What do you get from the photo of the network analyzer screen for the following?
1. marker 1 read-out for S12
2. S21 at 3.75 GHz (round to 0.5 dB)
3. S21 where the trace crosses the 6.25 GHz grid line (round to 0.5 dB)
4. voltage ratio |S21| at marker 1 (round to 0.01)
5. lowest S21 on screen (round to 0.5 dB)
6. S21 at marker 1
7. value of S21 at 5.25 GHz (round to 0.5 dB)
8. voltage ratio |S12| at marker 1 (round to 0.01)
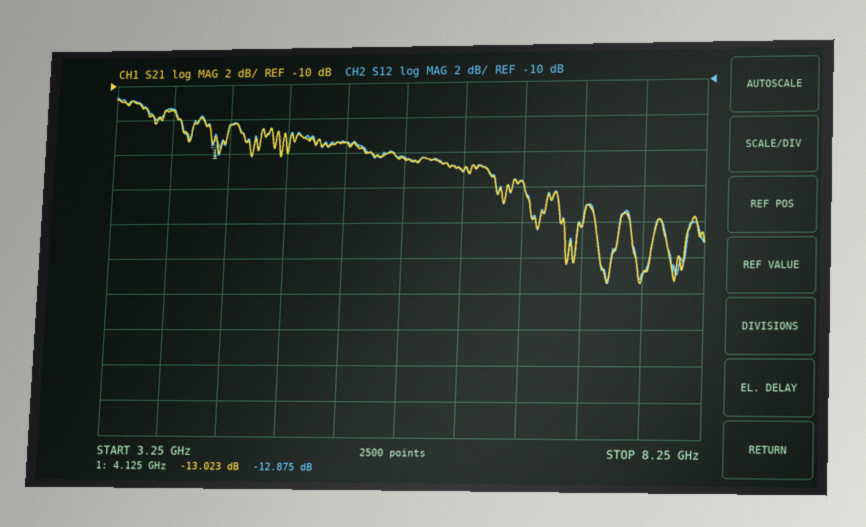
-12.875 dB
-11.5 dB
-15.0 dB
0.22
-21.5 dB
-13.023 dB
-13.5 dB
0.23
